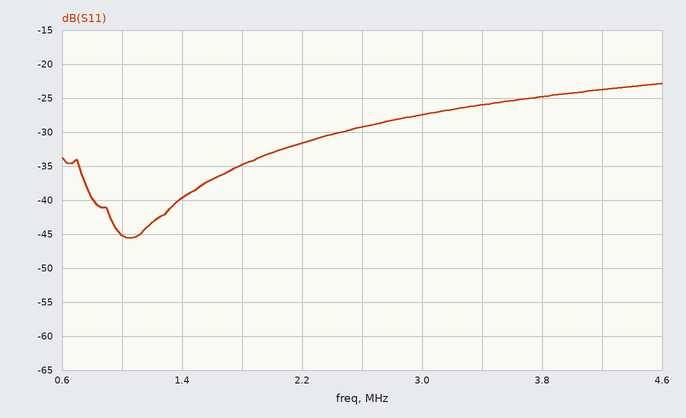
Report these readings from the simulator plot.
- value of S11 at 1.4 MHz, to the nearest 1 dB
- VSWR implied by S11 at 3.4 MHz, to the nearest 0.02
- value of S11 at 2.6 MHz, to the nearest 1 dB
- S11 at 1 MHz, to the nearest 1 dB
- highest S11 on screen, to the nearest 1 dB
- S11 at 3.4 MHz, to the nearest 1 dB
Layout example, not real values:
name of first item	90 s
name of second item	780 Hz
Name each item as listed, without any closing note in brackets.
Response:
value of S11 at 1.4 MHz, to the nearest 1 dB	-40 dB
VSWR implied by S11 at 3.4 MHz, to the nearest 0.02	1.10
value of S11 at 2.6 MHz, to the nearest 1 dB	-29 dB
S11 at 1 MHz, to the nearest 1 dB	-45 dB
highest S11 on screen, to the nearest 1 dB	-23 dB
S11 at 3.4 MHz, to the nearest 1 dB	-26 dB
